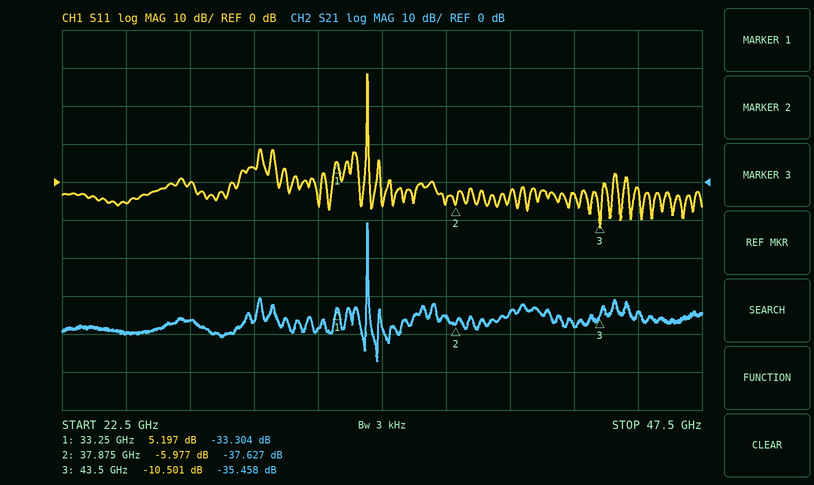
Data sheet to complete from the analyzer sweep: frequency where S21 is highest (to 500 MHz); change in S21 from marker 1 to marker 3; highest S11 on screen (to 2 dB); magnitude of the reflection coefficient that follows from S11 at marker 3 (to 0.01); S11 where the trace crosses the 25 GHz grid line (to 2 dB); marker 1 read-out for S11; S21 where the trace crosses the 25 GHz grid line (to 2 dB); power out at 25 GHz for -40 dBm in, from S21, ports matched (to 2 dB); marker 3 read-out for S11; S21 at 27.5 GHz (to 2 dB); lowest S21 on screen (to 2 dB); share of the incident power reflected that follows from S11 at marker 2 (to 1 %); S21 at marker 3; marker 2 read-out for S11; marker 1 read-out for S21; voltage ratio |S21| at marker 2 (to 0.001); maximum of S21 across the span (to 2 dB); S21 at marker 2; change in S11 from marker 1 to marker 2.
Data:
34.5 GHz
-2.154 dB
28 dB
0.30
-6 dB
5.197 dB
-40 dB
-80 dBm
-10.501 dB
-36 dB
-48 dB
25 %
-35.458 dB
-5.977 dB
-33.304 dB
0.013
-10 dB
-37.627 dB
-11.174 dB
